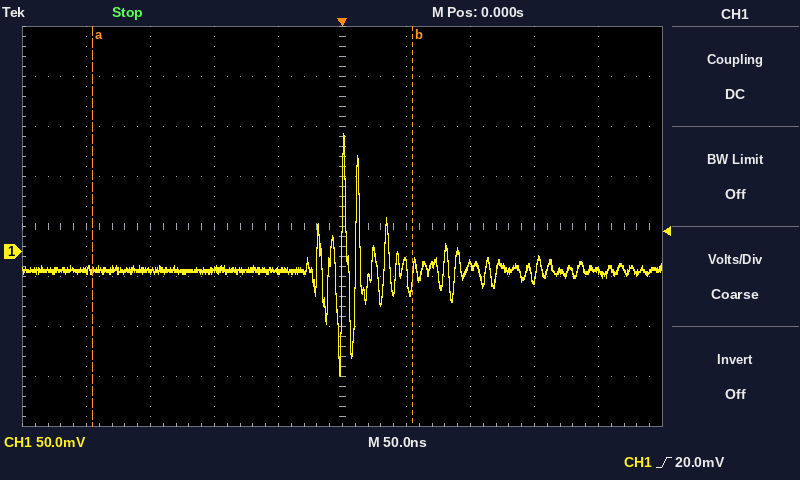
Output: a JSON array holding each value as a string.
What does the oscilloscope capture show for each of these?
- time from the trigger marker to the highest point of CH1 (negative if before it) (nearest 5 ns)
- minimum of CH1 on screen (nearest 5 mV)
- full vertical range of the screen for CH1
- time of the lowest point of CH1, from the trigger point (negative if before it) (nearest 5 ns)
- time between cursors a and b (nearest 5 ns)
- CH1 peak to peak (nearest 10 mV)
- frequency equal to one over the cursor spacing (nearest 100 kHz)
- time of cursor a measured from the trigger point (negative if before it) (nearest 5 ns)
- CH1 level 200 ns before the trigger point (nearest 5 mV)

["0 ns", "-125 mV", "400 mV", "0 ns", "250 ns", "240 mV", "4.0 MHz", "-195 ns", "-20 mV"]
